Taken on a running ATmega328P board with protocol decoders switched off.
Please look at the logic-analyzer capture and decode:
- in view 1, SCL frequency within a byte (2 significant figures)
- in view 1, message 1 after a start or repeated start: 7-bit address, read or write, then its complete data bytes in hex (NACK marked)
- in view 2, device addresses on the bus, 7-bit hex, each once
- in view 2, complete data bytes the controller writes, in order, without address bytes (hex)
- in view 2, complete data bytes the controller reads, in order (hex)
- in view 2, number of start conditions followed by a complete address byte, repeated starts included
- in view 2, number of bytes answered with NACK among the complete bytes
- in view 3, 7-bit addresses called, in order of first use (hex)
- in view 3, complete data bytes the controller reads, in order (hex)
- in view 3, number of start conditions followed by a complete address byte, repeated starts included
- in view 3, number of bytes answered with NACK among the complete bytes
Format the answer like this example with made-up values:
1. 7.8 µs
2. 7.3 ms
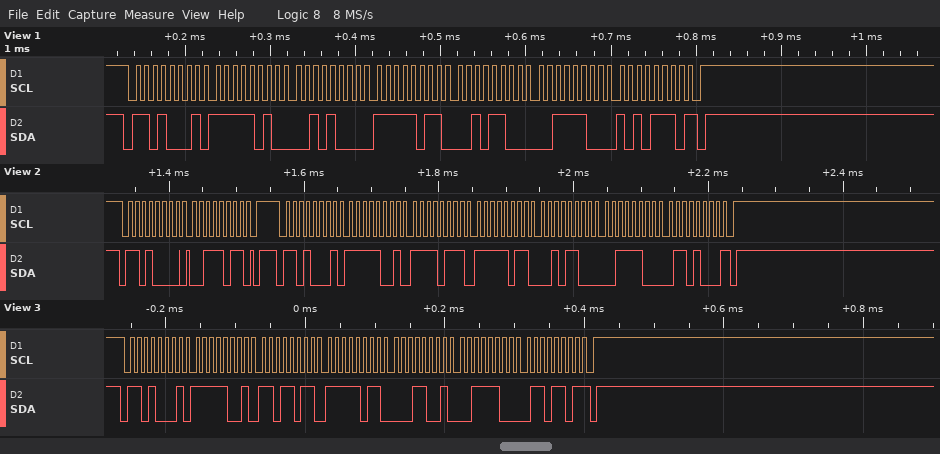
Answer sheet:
1. 100 kHz
2. 0x68 read: FA 28 FB 2C 3C AE NACK
3. 0x68
4. 3B
5. F9 F7 FB 2C 3C 68
6. 2
7. 1
8. 0x68
9. F9 DB FB 19 3C 6D
10. 1
11. 1
